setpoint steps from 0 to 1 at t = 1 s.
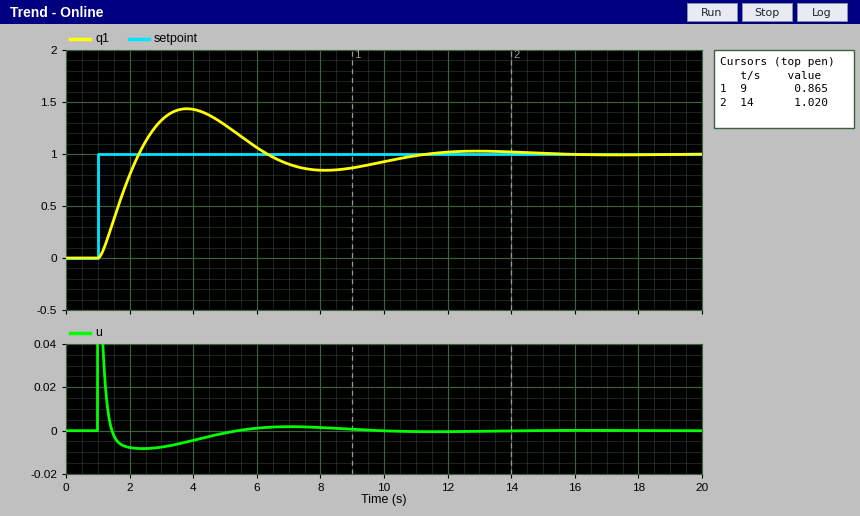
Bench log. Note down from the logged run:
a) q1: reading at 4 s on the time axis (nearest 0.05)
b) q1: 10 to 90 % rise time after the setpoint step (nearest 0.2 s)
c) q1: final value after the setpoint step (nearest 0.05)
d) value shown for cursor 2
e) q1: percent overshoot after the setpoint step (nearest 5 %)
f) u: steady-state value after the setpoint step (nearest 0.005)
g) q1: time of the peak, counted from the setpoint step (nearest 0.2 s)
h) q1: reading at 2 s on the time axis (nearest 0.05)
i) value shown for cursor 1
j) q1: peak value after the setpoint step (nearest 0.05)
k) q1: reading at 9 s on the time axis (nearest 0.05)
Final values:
1.45
1.0 s
1.00
1.020
45 %
0.000
2.8 s
0.80
0.865
1.45
0.85
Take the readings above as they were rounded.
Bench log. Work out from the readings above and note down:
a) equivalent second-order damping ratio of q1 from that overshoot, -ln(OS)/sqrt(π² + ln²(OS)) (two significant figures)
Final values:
0.25
